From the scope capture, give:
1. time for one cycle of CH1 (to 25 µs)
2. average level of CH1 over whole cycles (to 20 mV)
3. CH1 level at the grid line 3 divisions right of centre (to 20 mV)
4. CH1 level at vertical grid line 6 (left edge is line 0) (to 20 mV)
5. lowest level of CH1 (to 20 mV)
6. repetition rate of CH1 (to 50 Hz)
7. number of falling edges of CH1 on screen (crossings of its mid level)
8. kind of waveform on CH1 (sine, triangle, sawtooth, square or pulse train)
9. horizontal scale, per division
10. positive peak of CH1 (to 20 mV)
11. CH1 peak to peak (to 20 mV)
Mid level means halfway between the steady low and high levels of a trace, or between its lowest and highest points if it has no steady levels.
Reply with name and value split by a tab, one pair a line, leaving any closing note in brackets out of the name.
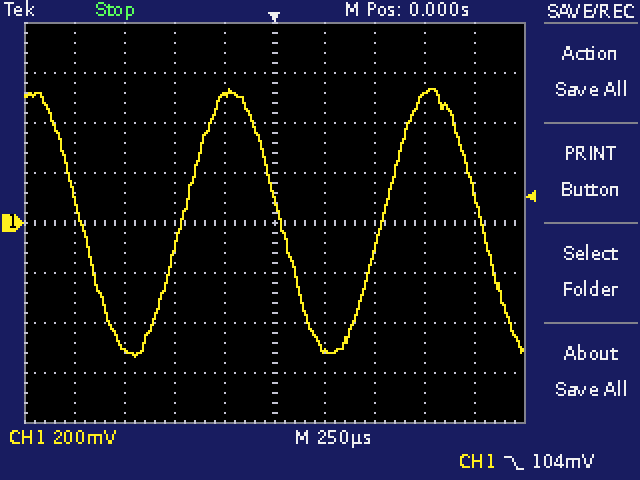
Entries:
time for one cycle of CH1	1.000 ms
average level of CH1 over whole cycles	0 mV
CH1 level at the grid line 3 divisions right of centre	520 mV
CH1 level at vertical grid line 6 (left edge is line 0)	-500 mV
lowest level of CH1	-540 mV
repetition rate of CH1	1.00 kHz
number of falling edges of CH1 on screen	3
kind of waveform on CH1	sine
horizontal scale, per division	250 µs
positive peak of CH1	540 mV
CH1 peak to peak	1.08 V
